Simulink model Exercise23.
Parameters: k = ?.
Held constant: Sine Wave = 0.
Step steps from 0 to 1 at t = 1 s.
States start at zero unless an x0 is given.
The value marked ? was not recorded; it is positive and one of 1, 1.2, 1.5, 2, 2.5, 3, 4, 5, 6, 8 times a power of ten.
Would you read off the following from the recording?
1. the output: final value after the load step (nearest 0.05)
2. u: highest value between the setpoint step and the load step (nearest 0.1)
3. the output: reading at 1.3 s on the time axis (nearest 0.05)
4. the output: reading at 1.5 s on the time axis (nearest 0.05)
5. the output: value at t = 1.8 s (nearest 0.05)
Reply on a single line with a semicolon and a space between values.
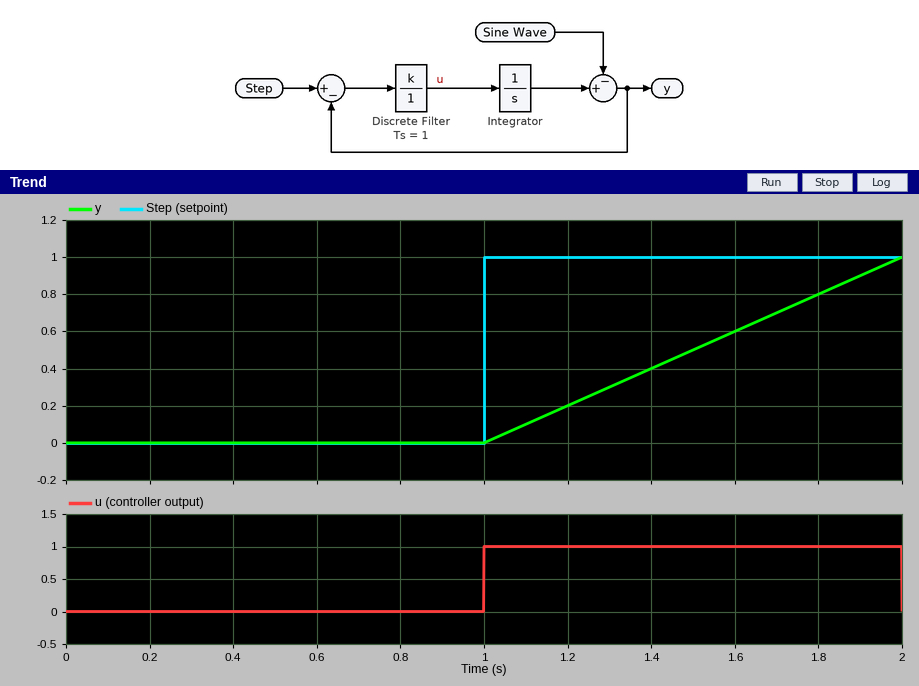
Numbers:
1.00; 1.0; 0.30; 0.50; 0.80
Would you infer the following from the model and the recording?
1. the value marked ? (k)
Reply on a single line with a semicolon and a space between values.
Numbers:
1
